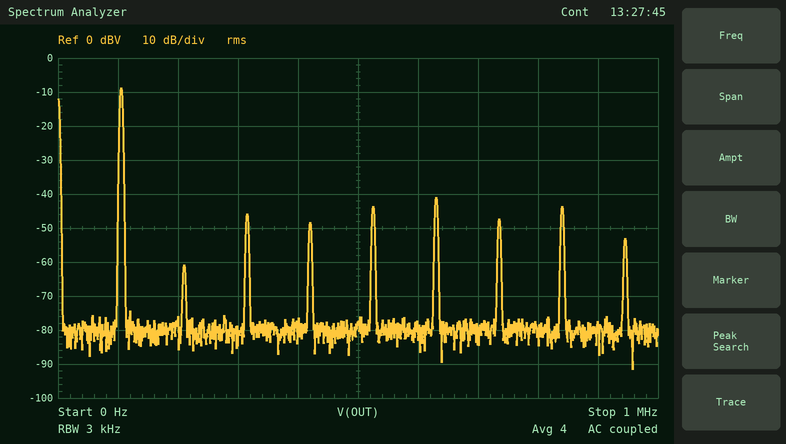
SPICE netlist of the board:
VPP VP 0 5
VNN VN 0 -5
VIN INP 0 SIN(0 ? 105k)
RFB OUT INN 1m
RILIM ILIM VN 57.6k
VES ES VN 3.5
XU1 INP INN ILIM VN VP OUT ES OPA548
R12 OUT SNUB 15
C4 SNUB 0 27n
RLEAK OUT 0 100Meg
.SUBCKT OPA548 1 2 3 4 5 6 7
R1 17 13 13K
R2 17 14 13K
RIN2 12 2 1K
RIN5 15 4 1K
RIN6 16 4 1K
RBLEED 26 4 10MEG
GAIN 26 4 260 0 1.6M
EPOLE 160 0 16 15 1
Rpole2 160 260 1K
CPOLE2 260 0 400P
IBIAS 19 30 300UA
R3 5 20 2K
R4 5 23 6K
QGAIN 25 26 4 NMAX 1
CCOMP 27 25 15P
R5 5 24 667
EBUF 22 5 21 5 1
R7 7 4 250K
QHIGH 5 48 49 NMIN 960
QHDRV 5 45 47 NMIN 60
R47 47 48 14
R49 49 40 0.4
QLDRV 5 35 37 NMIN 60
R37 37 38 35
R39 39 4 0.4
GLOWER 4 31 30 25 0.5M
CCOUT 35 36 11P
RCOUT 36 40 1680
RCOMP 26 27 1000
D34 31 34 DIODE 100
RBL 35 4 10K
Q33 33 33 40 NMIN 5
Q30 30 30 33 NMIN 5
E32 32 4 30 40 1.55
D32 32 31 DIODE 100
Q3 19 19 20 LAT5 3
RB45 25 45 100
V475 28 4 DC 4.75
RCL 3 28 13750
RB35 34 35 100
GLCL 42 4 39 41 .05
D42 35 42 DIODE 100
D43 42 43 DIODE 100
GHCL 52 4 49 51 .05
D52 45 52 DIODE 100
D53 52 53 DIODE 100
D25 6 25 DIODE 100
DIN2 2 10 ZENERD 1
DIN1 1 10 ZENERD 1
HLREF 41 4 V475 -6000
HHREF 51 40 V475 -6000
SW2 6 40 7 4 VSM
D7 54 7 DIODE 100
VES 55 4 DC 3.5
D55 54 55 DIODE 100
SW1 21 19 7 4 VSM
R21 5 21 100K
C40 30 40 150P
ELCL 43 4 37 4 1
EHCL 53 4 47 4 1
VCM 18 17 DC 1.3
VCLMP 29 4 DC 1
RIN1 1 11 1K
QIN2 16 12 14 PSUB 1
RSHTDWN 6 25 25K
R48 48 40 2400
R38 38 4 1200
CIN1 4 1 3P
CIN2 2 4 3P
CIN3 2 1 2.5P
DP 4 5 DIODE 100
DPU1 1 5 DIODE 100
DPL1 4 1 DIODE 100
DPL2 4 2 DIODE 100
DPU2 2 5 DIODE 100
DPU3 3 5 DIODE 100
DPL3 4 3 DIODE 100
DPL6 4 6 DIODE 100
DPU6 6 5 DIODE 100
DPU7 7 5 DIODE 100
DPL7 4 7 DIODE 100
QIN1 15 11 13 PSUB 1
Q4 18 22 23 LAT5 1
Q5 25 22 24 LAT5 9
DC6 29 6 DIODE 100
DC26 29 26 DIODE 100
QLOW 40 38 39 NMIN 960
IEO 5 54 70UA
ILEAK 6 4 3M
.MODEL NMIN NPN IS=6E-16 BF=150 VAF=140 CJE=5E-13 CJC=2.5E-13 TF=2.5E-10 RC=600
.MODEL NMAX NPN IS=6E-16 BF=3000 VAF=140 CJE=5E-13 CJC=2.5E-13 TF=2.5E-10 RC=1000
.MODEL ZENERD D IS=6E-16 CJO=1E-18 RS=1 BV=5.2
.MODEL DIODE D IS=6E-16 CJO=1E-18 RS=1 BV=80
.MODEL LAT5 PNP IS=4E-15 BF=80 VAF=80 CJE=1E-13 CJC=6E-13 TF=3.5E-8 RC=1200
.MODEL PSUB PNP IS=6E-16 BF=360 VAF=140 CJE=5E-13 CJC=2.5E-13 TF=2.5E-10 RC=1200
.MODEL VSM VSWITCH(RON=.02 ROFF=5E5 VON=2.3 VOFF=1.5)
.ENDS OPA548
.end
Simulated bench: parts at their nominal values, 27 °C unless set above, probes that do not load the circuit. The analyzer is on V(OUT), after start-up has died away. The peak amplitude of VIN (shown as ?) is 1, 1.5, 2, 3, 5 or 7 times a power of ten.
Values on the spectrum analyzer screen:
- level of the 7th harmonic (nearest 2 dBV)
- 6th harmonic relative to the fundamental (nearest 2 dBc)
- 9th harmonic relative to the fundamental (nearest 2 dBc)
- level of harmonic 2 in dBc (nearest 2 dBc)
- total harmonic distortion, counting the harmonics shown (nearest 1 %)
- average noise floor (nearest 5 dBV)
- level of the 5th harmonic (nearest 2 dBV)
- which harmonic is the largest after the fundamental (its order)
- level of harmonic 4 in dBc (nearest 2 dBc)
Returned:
-48 dBV
-32 dBc
-44 dBc
-52 dBc
4 %
-80 dBV
-44 dBV
6
-40 dBc
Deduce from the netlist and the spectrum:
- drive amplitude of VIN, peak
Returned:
500 mV
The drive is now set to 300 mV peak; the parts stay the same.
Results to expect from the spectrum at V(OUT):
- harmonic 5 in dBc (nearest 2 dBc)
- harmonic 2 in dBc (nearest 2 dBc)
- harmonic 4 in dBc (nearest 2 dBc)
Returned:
-44 dBc
-42 dBc
-34 dBc
